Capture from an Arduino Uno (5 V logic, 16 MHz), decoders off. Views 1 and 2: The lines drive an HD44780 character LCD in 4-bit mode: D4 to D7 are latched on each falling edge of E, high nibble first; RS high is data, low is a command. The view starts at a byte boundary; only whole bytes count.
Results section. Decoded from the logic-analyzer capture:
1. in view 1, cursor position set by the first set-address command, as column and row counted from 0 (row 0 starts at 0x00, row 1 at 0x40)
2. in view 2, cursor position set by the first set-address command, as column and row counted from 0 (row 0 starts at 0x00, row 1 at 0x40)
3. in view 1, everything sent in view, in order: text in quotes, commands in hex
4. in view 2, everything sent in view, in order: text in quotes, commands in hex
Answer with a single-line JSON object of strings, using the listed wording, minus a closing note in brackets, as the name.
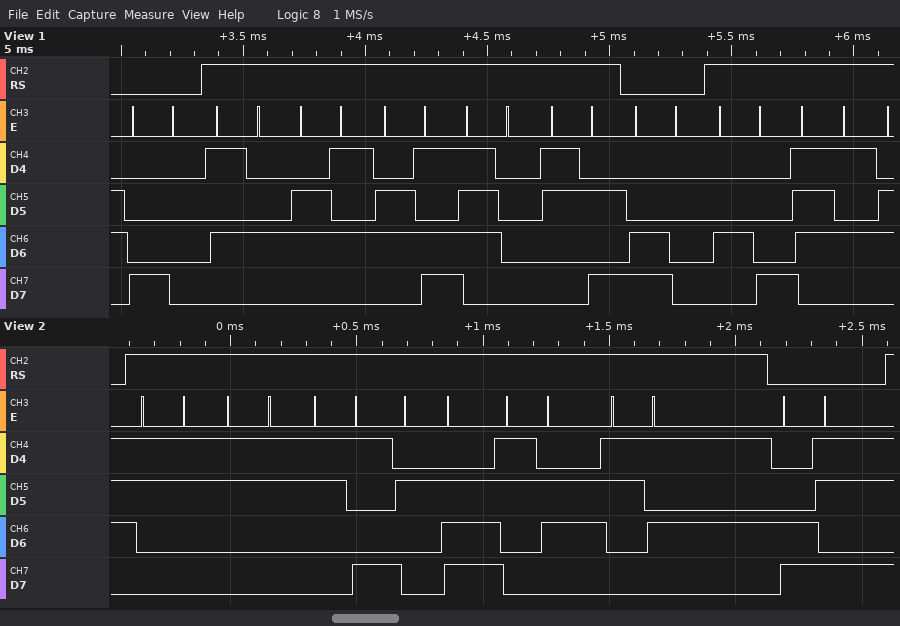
{"in view 1, cursor position set by the first set-address command, as column and row counted from 0": "column 0, row 0", "in view 2, cursor position set by the first set-address command, as column and row counted from 0": "column 11, row 1", "in view 1, everything sent in view, in order: text in quotes, commands in hex": "0x80 \"Temp:\" 0xC0 \"Hu\"", "in view 2, everything sent in view, in order: text in quotes, commands in hex": "\"339.65\" 0xCB"}
